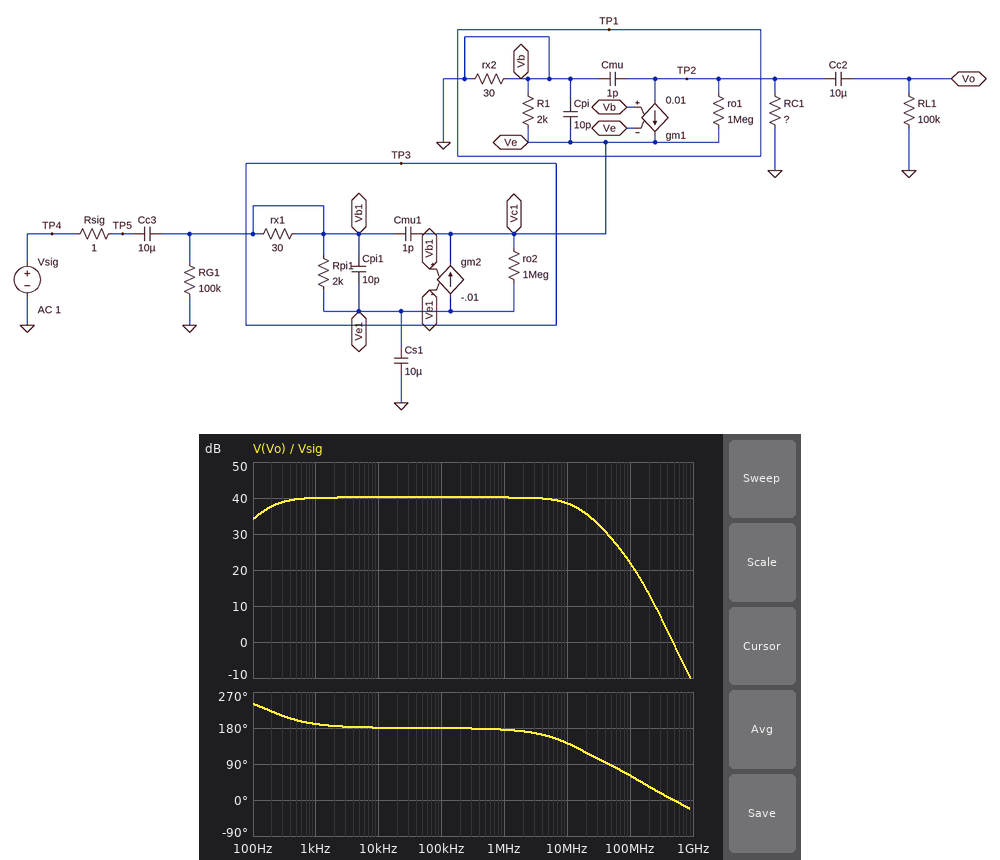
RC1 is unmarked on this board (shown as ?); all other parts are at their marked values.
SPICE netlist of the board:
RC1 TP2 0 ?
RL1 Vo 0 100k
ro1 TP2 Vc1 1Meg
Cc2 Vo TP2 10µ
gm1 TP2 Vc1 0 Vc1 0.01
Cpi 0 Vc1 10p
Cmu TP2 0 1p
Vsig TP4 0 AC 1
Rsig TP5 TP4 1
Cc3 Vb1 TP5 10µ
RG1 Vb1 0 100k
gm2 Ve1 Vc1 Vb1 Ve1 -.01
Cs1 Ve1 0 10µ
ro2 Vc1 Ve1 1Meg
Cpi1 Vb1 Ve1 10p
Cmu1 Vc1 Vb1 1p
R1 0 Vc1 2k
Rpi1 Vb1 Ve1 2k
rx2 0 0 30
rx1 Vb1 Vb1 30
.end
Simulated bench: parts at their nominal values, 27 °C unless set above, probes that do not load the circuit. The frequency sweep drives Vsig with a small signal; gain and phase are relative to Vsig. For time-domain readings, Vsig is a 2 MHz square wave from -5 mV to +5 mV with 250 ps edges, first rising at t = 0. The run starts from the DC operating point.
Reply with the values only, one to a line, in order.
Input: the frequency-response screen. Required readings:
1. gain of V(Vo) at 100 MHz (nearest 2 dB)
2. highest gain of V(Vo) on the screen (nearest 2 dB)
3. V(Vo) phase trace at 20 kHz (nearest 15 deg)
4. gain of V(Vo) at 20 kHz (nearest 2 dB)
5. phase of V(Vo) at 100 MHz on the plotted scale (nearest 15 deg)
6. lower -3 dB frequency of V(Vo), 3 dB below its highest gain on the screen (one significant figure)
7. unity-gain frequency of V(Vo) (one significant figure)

22 dB
40 dB
180 deg
40 dB
60 deg
200 Hz
500 MHz
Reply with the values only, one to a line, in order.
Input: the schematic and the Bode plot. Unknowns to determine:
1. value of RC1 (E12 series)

12 kΩ
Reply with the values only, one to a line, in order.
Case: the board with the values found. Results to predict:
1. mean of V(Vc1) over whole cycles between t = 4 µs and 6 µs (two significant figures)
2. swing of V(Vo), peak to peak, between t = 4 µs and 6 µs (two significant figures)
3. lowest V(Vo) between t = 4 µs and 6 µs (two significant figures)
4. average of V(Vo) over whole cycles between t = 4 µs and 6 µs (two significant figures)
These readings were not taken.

-4.8 mV
1.0 V
-1.0 V
-510 mV
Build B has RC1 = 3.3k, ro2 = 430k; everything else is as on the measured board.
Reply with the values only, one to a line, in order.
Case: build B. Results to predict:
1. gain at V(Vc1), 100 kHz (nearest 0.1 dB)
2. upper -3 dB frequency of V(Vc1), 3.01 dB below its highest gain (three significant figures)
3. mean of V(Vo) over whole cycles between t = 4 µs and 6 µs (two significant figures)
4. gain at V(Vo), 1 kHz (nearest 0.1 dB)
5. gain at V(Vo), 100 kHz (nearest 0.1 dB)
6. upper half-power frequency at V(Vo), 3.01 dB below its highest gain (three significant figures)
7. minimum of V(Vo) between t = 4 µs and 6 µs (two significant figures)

-0.4 dB
152 MHz
-150 mV
29.5 dB
29.7 dB
45.5 MHz
-300 mV
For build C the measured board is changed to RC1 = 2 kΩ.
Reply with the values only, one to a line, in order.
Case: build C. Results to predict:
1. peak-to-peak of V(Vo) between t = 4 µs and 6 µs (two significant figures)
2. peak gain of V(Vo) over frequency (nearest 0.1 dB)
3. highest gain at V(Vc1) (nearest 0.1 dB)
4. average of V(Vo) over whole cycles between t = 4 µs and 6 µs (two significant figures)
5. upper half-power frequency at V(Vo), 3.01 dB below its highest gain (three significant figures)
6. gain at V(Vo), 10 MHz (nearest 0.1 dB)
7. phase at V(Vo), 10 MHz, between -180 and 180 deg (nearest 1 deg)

190 mV
25.4 dB
-0.4 dB
-93 mV
66.8 MHz
25.3 dB
169 deg
